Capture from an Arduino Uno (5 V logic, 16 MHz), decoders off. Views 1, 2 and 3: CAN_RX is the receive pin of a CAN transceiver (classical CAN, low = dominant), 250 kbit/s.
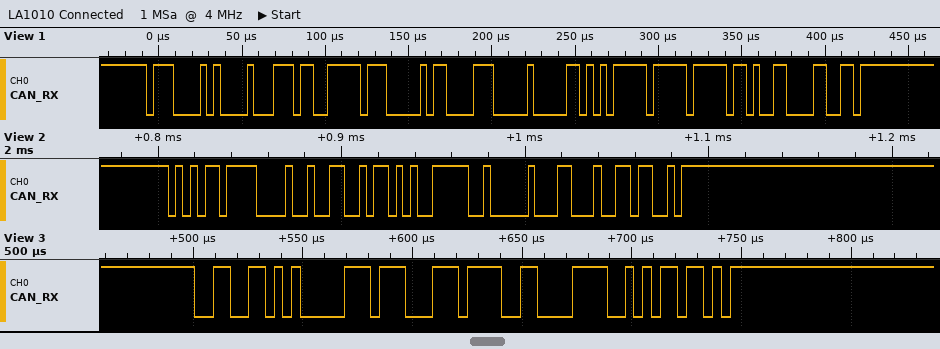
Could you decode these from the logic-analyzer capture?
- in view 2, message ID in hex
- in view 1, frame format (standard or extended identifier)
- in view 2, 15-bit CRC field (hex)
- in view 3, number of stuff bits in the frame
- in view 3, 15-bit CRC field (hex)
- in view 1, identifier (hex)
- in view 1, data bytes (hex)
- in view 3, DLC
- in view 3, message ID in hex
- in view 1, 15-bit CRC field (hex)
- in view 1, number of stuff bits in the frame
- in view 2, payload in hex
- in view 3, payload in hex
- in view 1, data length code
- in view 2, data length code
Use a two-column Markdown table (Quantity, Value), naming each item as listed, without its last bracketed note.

| Quantity | Value |
|---|---|
| in view 2, message ID in hex | 0x56F |
| in view 1, frame format | standard |
| in view 2, 15-bit CRC field | 0x626C |
| in view 3, number of stuff bits in the frame | 1 |
| in view 3, 15-bit CRC field | 0x72B6 |
| in view 1, identifier | 0x70A |
| in view 1, data bytes | EC FF 03 0E 00 55 FF FF |
| in view 3, DLC | 3 |
| in view 3, message ID in hex | 0x335 |
| in view 1, 15-bit CRC field | 0x2619 |
| in view 1, number of stuff bits in the frame | 7 |
| in view 2, payload in hex | 99 6A 7D 00 |
| in view 3, payload in hex | 71 DE 61 |
| in view 1, data length code | 8 |
| in view 2, data length code | 4 |
